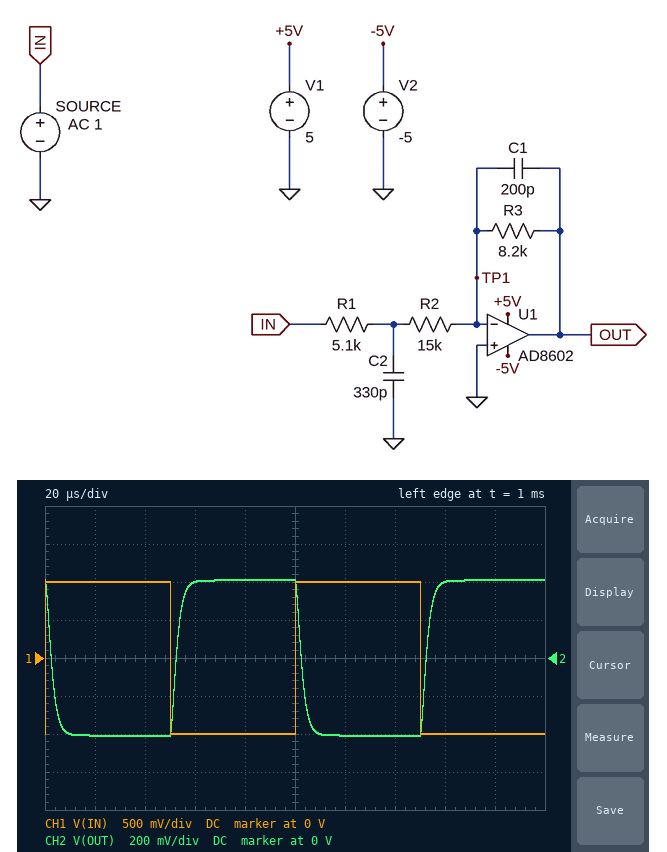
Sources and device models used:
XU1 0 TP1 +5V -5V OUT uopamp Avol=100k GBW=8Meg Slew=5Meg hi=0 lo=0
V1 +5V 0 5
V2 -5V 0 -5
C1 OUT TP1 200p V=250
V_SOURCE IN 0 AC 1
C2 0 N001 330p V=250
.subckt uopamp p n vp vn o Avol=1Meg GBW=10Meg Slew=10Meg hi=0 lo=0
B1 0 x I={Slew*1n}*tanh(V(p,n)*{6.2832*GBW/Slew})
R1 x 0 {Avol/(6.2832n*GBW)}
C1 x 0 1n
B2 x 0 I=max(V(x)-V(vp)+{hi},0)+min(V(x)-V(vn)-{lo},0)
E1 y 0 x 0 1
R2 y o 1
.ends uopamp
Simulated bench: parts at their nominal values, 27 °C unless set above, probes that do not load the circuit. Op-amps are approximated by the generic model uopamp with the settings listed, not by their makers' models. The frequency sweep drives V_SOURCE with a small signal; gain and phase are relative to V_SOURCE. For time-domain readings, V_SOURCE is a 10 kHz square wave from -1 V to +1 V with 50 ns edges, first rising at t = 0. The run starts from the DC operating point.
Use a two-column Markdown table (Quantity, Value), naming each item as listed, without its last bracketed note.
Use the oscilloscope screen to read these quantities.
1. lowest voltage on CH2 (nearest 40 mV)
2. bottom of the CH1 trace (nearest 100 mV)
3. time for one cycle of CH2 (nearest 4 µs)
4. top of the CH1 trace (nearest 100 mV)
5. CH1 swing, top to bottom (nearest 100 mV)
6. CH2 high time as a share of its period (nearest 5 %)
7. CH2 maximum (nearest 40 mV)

| Quantity | Value |
|---|---|
| lowest voltage on CH2 | -400 mV |
| bottom of the CH1 trace | -1.0 V |
| time for one cycle of CH2 | 100 µs |
| top of the CH1 trace | 1.0 V |
| CH1 swing, top to bottom | 2.0 V |
| CH2 high time as a share of its period | 50 % |
| CH2 maximum | 400 mV |
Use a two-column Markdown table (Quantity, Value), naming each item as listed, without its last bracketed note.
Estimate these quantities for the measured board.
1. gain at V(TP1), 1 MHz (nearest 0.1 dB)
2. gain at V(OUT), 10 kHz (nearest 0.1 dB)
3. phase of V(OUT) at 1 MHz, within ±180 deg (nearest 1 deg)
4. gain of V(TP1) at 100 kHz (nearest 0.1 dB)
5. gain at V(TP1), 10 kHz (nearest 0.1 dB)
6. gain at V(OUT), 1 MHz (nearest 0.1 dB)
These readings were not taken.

| Quantity | Value |
|---|---|
| gain at V(TP1), 1 MHz | -64.3 dB |
| gain at V(OUT), 10 kHz | -7.9 dB |
| phase of V(OUT) at 1 MHz, within ±180 deg | 6 deg |
| gain of V(TP1) at 100 kHz | -51.1 dB |
| gain at V(TP1), 10 kHz | -65.9 dB |
| gain at V(OUT), 1 MHz | -46.2 dB |
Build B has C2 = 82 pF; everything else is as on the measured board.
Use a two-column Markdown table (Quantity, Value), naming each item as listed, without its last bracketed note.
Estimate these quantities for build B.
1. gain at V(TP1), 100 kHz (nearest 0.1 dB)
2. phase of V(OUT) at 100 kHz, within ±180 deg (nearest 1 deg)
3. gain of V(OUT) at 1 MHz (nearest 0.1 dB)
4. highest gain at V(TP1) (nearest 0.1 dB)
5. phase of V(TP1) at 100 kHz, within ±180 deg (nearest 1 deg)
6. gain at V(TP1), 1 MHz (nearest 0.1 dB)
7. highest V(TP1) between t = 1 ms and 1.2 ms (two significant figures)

| Quantity | Value |
|---|---|
| gain at V(TP1), 100 kHz | -49.2 dB |
| phase of V(OUT) at 100 kHz, within ±180 deg | 122 deg |
| gain of V(OUT) at 1 MHz | -35.1 dB |
| highest gain at V(TP1) | -47.7 dB |
| phase of V(TP1) at 100 kHz, within ±180 deg | 32 deg |
| gain at V(TP1), 1 MHz | -53.1 dB |
| highest V(TP1) between t = 1 ms and 1.2 ms | 6.7 mV |
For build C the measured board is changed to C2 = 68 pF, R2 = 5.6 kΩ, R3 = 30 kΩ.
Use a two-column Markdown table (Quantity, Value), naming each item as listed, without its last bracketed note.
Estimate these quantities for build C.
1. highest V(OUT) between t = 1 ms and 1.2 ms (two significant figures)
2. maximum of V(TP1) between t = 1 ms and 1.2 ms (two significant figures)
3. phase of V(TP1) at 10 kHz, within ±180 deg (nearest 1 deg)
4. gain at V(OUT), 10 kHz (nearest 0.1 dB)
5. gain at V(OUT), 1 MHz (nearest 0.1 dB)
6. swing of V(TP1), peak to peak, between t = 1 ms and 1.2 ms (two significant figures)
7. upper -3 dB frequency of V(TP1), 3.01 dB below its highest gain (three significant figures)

| Quantity | Value |
|---|---|
| highest V(OUT) between t = 1 ms and 1.2 ms | 2.8 V |
| maximum of V(TP1) between t = 1 ms and 1.2 ms | 17 mV |
| phase of V(TP1) at 10 kHz, within ±180 deg | 68 deg |
| gain at V(OUT), 10 kHz | 8.4 dB |
| gain at V(OUT), 1 MHz | -26.4 dB |
| swing of V(TP1), peak to peak, between t = 1 ms and 1.2 ms | 33 mV |
| upper -3 dB frequency of V(TP1), 3.01 dB below its highest gain | 909 kHz |
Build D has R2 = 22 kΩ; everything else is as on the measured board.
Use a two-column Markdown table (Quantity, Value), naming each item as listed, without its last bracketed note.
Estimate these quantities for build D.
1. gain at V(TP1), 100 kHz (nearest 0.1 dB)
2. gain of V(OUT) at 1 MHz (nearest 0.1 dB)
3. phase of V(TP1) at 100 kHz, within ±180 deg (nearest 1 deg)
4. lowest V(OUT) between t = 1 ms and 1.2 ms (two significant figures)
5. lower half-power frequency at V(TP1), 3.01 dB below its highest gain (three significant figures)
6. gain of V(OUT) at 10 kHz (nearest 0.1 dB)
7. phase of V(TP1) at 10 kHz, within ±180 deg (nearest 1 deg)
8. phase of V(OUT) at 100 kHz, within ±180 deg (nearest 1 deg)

| Quantity | Value |
|---|---|
| gain at V(TP1), 100 kHz | -54.0 dB |
| gain of V(OUT) at 1 MHz | -49.5 dB |
| phase of V(TP1) at 100 kHz, within ±180 deg | 3 deg |
| lowest V(OUT) between t = 1 ms and 1.2 ms | -300 mV |
| lower half-power frequency at V(TP1), 3.01 dB below its highest gain | 43.8 kHz |
| gain of V(OUT) at 10 kHz | -10.5 dB |
| phase of V(TP1) at 10 kHz, within ±180 deg | 79 deg |
| phase of V(OUT) at 100 kHz, within ±180 deg | 93 deg |
